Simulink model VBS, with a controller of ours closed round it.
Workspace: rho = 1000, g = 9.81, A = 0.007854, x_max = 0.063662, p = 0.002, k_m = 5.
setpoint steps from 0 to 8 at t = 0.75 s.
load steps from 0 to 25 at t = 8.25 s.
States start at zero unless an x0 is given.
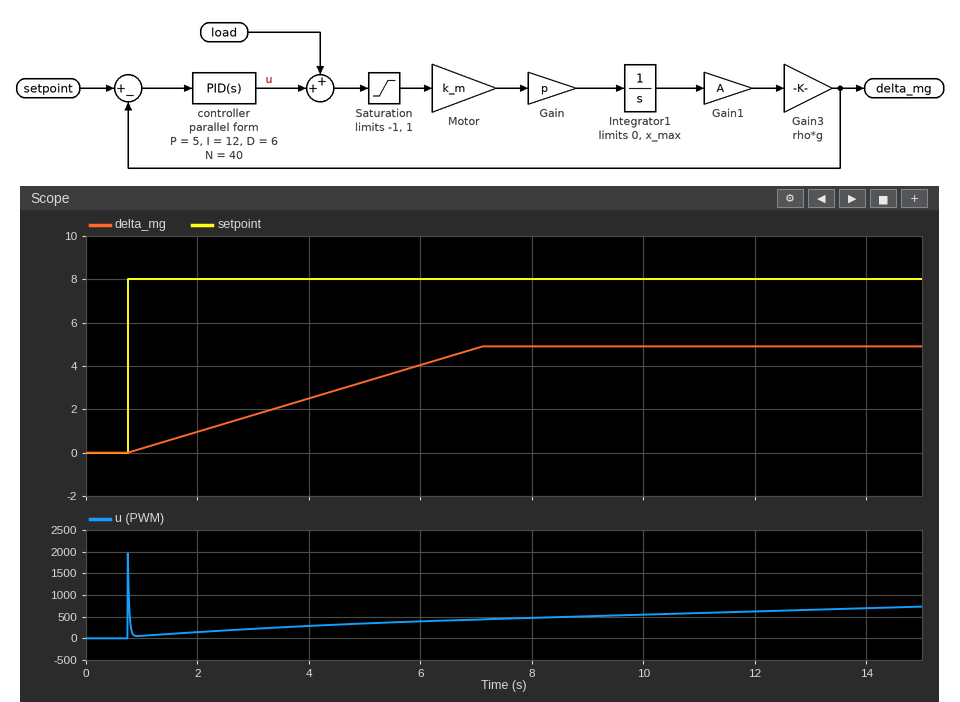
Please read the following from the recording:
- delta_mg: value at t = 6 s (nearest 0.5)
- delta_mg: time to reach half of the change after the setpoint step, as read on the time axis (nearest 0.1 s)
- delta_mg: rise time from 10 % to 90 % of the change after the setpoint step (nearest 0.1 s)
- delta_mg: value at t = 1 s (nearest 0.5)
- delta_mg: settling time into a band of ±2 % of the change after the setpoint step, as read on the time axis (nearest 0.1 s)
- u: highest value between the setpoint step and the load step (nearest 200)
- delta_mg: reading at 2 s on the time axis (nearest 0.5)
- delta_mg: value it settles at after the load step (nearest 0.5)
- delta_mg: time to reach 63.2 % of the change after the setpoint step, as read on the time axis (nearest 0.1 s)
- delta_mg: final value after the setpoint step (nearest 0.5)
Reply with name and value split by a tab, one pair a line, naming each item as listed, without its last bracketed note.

delta_mg: value at t = 6 s	4.0
delta_mg: time to reach half of the change after the setpoint step, as read on the time axis	3.9 s
delta_mg: rise time from 10 % to 90 % of the change after the setpoint step	5.1 s
delta_mg: value at t = 1 s	0.0
delta_mg: settling time into a band of ±2 % of the change after the setpoint step, as read on the time axis	7.0 s
u: highest value between the setpoint step and the load step	2000
delta_mg: reading at 2 s on the time axis	1.0
delta_mg: value it settles at after the load step	5.0
delta_mg: time to reach 63.2 % of the change after the setpoint step, as read on the time axis	4.8 s
delta_mg: final value after the setpoint step	5.0
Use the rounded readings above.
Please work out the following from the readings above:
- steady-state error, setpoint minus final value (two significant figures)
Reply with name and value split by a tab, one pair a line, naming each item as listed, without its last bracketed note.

steady-state error, setpoint minus final value	3.0
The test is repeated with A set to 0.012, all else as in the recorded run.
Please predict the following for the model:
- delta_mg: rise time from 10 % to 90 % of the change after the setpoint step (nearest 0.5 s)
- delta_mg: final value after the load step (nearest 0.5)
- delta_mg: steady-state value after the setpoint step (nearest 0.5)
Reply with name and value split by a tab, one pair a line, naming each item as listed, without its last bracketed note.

delta_mg: rise time from 10 % to 90 % of the change after the setpoint step	5.0 s
delta_mg: final value after the load step	7.5
delta_mg: steady-state value after the setpoint step	7.5
